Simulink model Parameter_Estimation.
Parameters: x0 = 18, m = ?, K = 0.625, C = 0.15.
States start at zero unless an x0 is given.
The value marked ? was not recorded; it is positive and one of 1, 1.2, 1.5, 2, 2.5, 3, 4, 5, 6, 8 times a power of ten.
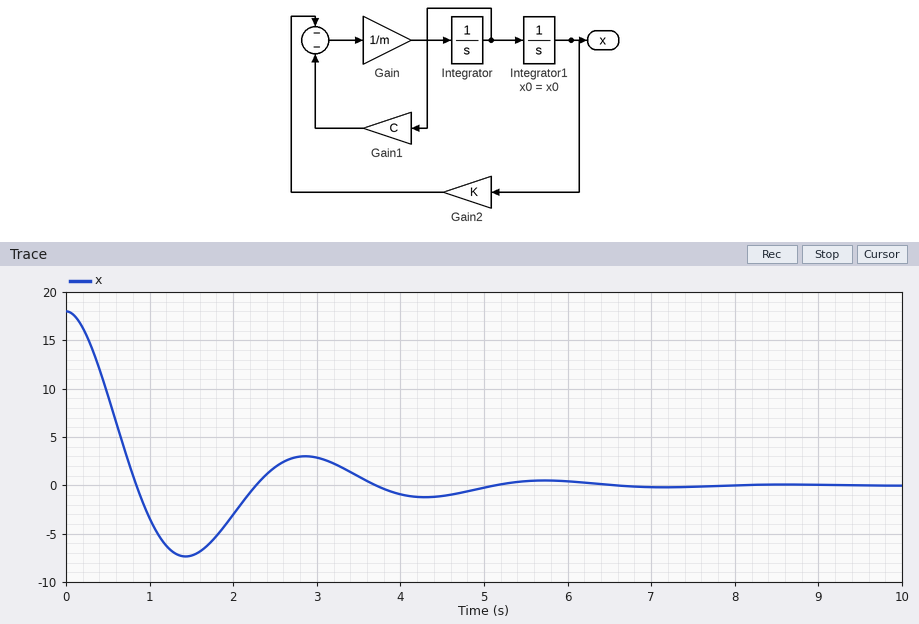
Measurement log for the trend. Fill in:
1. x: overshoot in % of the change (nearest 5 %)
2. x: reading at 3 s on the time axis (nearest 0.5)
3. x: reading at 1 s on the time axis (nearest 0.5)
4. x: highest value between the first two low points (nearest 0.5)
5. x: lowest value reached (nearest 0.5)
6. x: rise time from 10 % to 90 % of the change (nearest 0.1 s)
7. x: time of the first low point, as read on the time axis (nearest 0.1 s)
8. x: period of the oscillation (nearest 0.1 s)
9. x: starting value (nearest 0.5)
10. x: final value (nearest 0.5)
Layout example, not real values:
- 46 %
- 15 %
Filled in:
- 40 %
- 3.0
- -3.5
- 3.0
- -7.5
- 0.6 s
- 1.4 s
- 2.9 s
- 18.0
- 0.0
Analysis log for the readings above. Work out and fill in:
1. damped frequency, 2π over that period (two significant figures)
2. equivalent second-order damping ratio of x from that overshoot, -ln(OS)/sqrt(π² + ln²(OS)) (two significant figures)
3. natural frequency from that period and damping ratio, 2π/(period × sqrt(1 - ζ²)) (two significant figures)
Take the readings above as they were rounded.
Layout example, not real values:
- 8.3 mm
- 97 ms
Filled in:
- 2.2 rad/s
- 0.28
- 2.3 rad/s
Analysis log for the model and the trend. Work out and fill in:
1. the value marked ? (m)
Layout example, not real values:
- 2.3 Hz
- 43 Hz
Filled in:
- 0.12
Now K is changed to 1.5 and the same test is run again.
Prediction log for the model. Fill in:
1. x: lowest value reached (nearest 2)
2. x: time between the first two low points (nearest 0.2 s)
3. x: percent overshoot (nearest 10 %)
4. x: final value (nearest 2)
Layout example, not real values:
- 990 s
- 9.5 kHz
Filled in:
- -10
- 1.8 s
- 60 %
- 0
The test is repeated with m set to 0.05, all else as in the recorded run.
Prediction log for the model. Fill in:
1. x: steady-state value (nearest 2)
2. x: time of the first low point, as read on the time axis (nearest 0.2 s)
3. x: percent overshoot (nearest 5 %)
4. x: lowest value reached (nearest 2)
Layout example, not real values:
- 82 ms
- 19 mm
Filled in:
- 0
- 1.0 s
- 25 %
- -4
